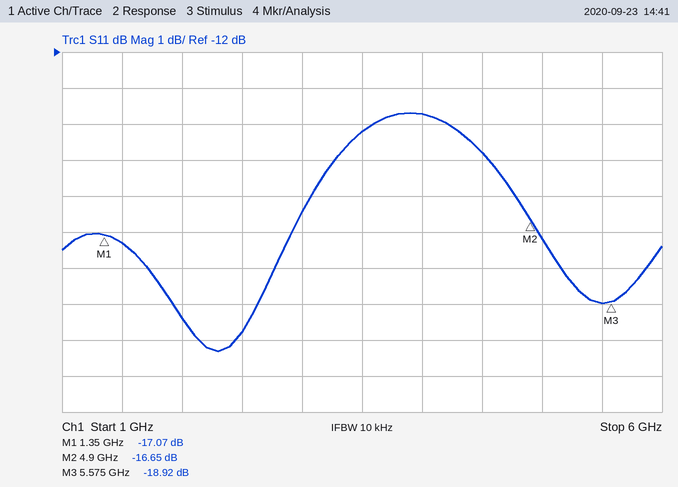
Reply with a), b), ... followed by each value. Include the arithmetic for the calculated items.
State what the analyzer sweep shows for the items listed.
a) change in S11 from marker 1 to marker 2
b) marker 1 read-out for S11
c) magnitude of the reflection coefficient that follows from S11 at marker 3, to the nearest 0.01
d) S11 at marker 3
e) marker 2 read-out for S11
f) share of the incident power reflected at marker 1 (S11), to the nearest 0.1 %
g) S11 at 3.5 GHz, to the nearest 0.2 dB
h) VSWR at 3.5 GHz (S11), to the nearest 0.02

a) -16.65 − (-17.07) = 0.42 dB
b) -17.07 dB
c) 10^(-18.92/20) ≈ 0.11
d) -18.92 dB
e) -16.65 dB
f) 10^(-17.07/10) ≈ 2.0 %
g) -14.2 dB
h) |Γ| = 10^(-14.2/20) = 0.1950; VSWR = (1 + 0.1950)/(1 − 0.1950) ≈ 1.48
